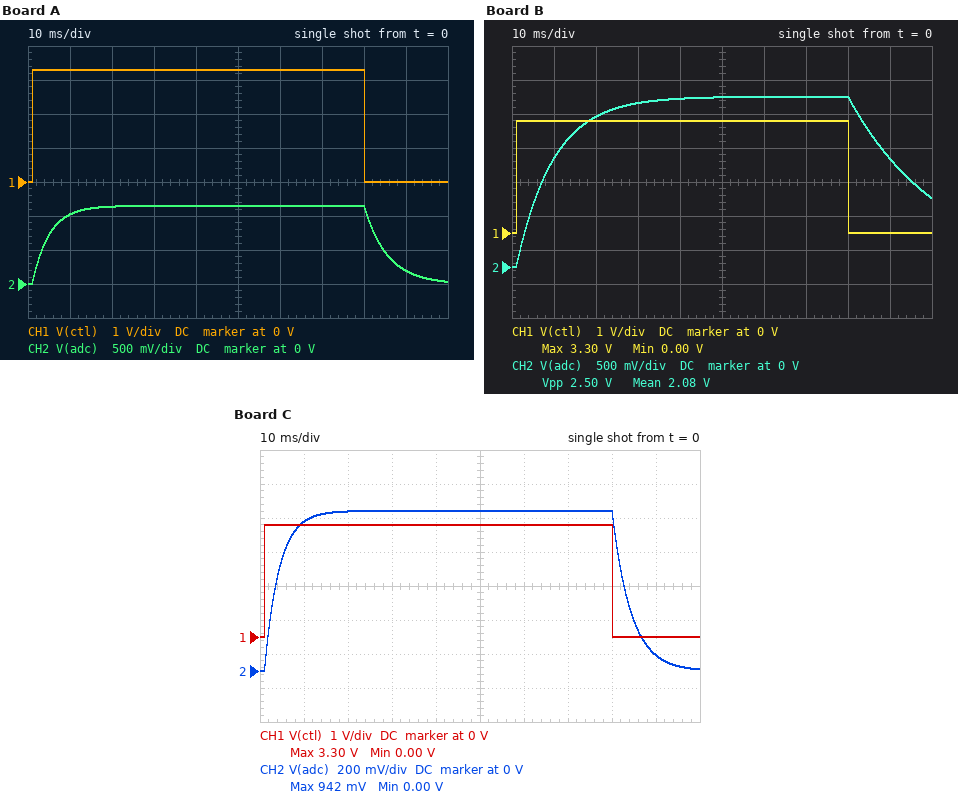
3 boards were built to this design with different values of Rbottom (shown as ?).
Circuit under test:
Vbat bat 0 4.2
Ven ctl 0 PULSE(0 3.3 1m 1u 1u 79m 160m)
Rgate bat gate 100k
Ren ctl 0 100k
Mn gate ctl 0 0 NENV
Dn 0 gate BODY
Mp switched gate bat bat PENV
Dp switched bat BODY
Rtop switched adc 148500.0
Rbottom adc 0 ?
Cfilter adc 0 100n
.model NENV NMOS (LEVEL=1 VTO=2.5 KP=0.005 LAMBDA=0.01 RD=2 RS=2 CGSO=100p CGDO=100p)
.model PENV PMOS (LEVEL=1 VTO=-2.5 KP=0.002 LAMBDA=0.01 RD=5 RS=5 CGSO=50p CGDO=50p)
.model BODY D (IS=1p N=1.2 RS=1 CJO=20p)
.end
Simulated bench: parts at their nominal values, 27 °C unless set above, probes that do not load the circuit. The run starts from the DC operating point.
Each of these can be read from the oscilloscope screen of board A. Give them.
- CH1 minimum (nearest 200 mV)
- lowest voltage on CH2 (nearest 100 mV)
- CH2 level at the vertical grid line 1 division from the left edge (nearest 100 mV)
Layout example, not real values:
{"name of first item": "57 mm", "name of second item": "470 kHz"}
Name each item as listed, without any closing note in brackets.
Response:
{"CH1 minimum": "0 V", "lowest voltage on CH2": "0 V", "CH2 level at the vertical grid line 1 division from the left edge": "1.0 V"}
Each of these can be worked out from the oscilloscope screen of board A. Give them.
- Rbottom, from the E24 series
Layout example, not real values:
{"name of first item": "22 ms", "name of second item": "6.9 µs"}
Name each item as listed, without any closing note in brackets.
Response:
{"Rbottom, from the E24 series": "56 kΩ"}
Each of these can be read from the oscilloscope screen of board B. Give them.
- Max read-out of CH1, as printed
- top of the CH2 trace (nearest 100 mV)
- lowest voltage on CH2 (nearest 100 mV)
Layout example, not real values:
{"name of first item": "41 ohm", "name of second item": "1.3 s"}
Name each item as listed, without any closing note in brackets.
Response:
{"Max read-out of CH1, as printed": "3.30 V", "top of the CH2 trace": "2.5 V", "lowest voltage on CH2": "0 V"}
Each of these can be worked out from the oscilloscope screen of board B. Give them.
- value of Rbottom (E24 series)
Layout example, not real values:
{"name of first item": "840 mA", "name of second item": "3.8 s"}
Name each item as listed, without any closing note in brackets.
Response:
{"value of Rbottom": "220 kΩ"}
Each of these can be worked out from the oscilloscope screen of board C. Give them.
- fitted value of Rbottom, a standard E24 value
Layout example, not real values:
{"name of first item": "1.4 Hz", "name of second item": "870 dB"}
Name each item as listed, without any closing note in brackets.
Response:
{"fitted value of Rbottom, a standard E24 value": "43 kΩ"}
